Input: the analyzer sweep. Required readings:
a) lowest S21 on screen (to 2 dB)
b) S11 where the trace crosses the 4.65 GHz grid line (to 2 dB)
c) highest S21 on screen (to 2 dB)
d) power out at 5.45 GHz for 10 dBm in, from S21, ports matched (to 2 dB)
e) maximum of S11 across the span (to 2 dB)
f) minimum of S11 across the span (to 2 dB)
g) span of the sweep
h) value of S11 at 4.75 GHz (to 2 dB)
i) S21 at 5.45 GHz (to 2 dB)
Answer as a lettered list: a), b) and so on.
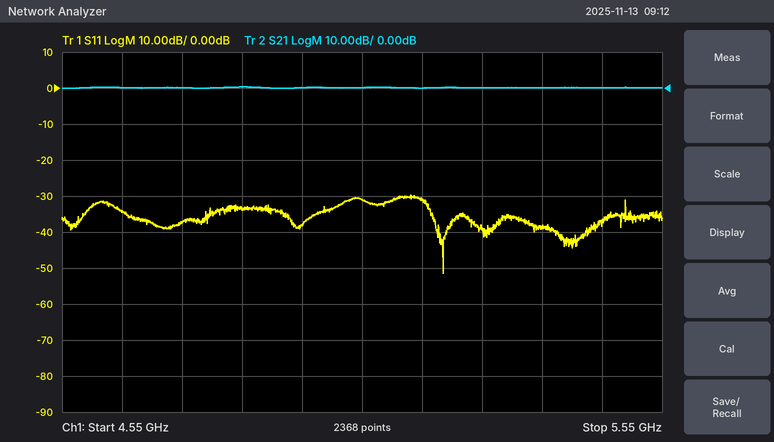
a) 0 dB
b) -34 dB
c) 0 dB
d) 10 dBm
e) -30 dB
f) -52 dB
g) 1 GHz
h) -38 dB
i) 0 dB
